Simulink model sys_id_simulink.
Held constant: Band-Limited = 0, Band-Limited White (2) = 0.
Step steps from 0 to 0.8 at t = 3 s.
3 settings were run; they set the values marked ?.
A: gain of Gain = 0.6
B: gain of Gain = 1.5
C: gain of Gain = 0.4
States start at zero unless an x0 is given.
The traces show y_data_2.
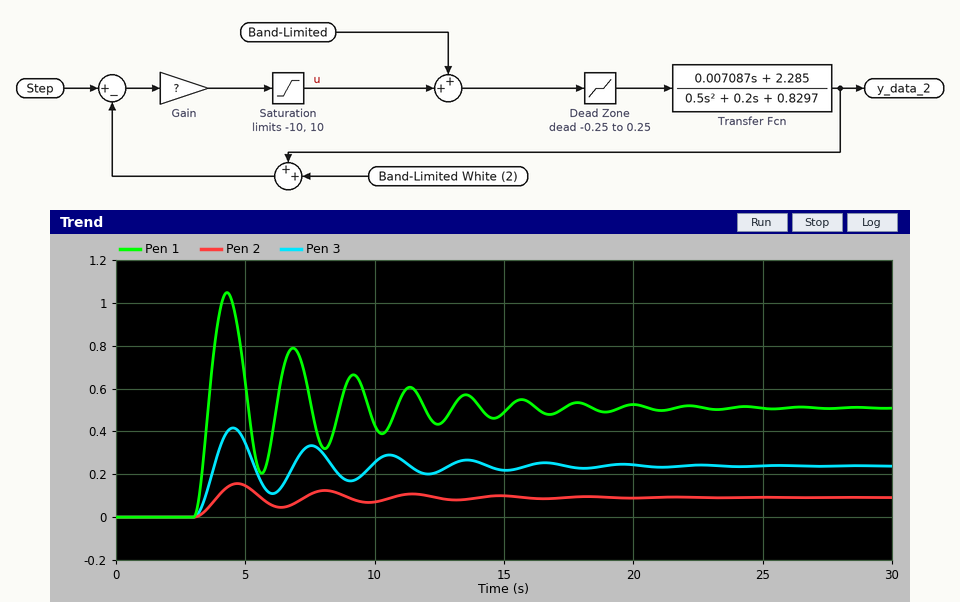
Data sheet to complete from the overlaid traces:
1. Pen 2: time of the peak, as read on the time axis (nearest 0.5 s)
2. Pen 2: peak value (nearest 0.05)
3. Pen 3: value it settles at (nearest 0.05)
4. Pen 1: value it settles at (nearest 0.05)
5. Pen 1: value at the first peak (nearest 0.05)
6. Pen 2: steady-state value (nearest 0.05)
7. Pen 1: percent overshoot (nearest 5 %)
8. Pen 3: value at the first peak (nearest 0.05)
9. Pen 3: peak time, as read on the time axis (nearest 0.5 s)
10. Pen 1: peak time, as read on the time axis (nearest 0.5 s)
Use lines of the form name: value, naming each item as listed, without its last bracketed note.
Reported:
Pen 2: time of the peak, as read on the time axis: 4.5 s
Pen 2: peak value: 0.15
Pen 3: value it settles at: 0.25
Pen 1: value it settles at: 0.50
Pen 1: value at the first peak: 1.05
Pen 2: steady-state value: 0.10
Pen 1: percent overshoot: 105 %
Pen 3: value at the first peak: 0.40
Pen 3: peak time, as read on the time axis: 4.5 s
Pen 1: peak time, as read on the time axis: 4.5 s
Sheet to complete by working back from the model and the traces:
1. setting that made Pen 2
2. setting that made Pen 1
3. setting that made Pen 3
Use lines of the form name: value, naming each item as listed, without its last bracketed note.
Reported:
setting that made Pen 2: C
setting that made Pen 1: B
setting that made Pen 3: A
